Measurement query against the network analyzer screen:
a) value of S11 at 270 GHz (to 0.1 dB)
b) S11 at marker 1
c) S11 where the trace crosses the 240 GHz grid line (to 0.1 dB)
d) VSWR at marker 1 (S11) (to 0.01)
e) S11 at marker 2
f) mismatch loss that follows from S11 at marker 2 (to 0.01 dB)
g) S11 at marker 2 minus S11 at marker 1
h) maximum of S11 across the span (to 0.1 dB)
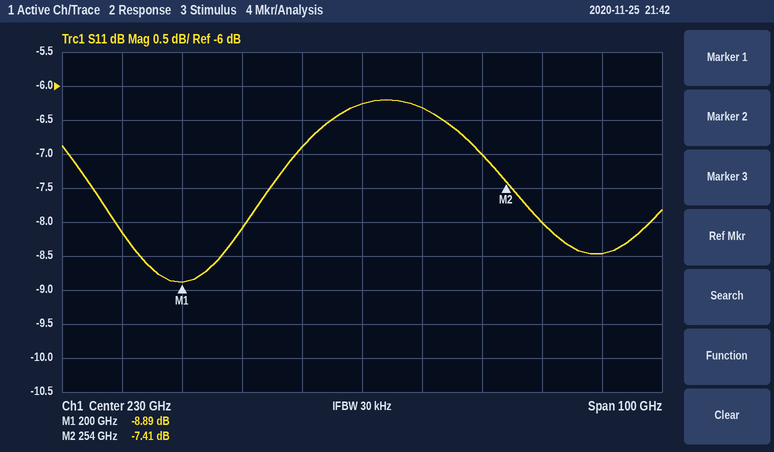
-8.5 dB
-8.89 dB
-6.3 dB
2.12
-7.41 dB
0.87 dB
1.48 dB
-6.2 dB
